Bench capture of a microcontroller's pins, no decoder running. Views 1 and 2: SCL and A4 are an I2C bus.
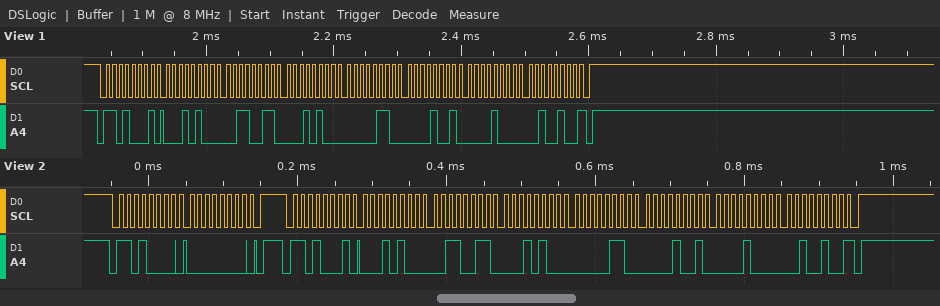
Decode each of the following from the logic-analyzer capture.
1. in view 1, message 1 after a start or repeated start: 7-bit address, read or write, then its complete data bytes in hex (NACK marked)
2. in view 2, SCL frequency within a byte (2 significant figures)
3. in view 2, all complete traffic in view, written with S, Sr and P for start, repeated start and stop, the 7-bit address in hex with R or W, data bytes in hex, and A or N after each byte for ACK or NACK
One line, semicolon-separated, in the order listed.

0x68 read: 14 33 14 06 09 08 24 NACK; 100 kHz; S 68W A 00 A P S 68R A 14 A 33 A 14 A 06 A 09 A 08 A 24 N P
